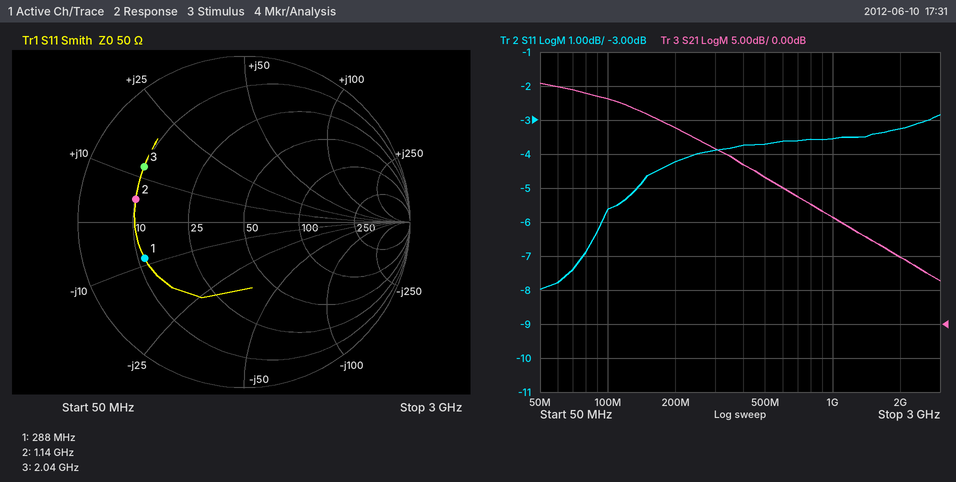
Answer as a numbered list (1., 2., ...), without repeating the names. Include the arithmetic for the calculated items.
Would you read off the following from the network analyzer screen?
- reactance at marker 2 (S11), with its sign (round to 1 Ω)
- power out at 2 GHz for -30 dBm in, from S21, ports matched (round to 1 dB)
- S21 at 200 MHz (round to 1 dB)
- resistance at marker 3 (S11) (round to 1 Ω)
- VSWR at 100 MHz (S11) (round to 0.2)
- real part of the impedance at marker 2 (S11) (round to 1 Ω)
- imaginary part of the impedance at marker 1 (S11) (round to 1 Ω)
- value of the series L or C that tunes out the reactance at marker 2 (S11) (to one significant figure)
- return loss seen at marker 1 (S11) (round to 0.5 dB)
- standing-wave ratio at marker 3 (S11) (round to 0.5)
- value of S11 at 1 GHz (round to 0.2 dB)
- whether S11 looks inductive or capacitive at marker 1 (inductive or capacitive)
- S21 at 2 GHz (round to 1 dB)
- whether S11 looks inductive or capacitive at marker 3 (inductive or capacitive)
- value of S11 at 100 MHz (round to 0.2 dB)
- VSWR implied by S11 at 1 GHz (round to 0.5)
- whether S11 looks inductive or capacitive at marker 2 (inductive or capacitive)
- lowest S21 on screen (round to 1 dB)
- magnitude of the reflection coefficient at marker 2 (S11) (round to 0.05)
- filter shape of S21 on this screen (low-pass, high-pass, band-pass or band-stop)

1. +5 Ω
2. -30 dBm + (10 dB) = -20 dBm
3. 29 dB
4. 10 Ω
5. |Γ| = 10^(-5.6/20) = 0.5248; VSWR = (1 + 0.5248)/(1 − 0.5248) ≈ 3.2
6. 10 Ω
7. -8 Ω
8. C = 1/(2π × 1.14 GHz × 5 Ω) ≈ 27.9 pF, so 30 pF to one significant figure
9. 4.0 dB
10. 5.5
11. -3.6 dB
12. capacitive
13. 10 dB
14. inductive
15. -5.6 dB
16. |Γ| = 10^(-3.6/20) = 0.6607; VSWR = (1 + 0.6607)/(1 − 0.6607) ≈ 4.89, so 5.0 to the nearest 0.5
17. inductive
18. 6 dB
19. 0.65
20. low-pass
